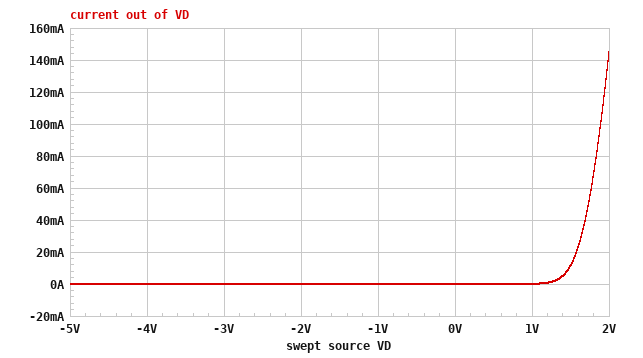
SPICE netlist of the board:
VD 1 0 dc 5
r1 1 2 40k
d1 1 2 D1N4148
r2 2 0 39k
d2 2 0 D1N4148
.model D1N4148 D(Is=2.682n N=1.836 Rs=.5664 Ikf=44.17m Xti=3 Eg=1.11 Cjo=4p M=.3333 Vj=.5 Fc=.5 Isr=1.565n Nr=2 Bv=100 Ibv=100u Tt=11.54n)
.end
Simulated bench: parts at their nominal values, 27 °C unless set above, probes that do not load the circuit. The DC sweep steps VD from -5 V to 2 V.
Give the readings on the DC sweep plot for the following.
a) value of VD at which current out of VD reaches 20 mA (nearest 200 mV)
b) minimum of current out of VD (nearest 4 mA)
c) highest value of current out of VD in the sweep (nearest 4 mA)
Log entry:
1.6 V
0 A
144 mA
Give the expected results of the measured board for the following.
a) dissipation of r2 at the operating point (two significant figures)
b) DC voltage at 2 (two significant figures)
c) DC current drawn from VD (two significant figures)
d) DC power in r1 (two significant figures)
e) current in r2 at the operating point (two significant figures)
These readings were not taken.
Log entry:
160 µW
2.5 V
2.4 A
160 µW
64 µA
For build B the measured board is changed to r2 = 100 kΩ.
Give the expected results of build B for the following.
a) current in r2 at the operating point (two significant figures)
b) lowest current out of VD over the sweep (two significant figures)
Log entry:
25 µA
-36 µA
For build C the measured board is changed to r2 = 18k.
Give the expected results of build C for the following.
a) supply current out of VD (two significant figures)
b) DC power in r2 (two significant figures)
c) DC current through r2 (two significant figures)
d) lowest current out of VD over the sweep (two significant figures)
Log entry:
2.4 A
350 µW
140 µA
-86 µA
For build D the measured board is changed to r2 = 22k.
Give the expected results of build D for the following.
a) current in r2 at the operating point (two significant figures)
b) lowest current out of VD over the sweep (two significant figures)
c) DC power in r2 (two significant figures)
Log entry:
110 µA
-81 µA
280 µW
